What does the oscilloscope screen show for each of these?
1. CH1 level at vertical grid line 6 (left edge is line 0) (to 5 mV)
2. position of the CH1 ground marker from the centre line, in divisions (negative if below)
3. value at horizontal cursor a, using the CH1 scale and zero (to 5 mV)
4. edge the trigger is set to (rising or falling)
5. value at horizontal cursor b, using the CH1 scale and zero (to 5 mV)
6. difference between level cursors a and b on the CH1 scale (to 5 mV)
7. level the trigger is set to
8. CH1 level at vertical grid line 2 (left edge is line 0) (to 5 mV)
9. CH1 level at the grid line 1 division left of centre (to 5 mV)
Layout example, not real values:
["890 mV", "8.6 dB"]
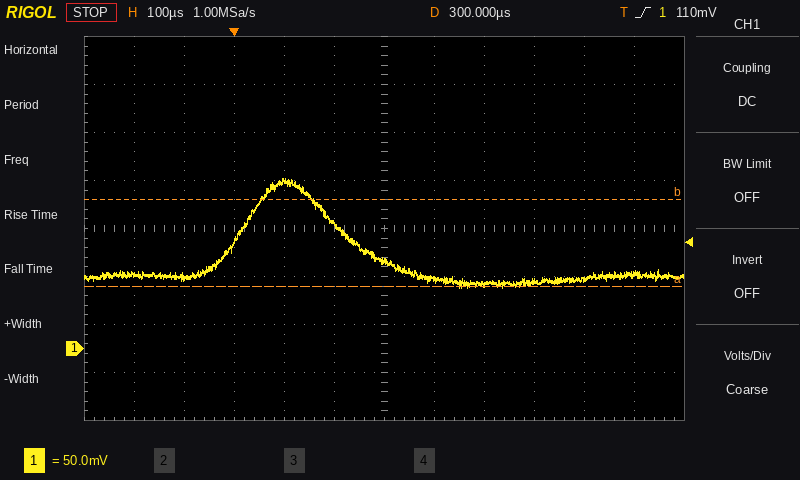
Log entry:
["90 mV", "-2.5 div", "65 mV", "rising", "155 mV", "90 mV", "110 mV", "75 mV", "130 mV"]
